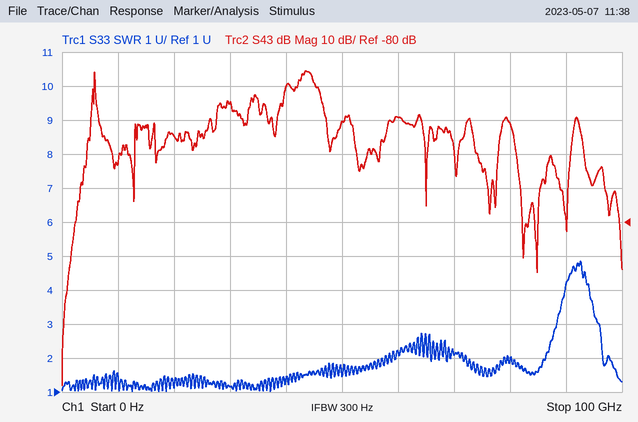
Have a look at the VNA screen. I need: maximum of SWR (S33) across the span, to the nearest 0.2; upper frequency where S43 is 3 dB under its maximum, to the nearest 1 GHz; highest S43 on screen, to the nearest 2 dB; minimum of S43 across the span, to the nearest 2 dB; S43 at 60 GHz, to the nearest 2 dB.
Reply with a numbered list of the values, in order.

1. 4.8
2. 45 GHz
3. -36 dB
4. -128 dB
5. -50 dB
